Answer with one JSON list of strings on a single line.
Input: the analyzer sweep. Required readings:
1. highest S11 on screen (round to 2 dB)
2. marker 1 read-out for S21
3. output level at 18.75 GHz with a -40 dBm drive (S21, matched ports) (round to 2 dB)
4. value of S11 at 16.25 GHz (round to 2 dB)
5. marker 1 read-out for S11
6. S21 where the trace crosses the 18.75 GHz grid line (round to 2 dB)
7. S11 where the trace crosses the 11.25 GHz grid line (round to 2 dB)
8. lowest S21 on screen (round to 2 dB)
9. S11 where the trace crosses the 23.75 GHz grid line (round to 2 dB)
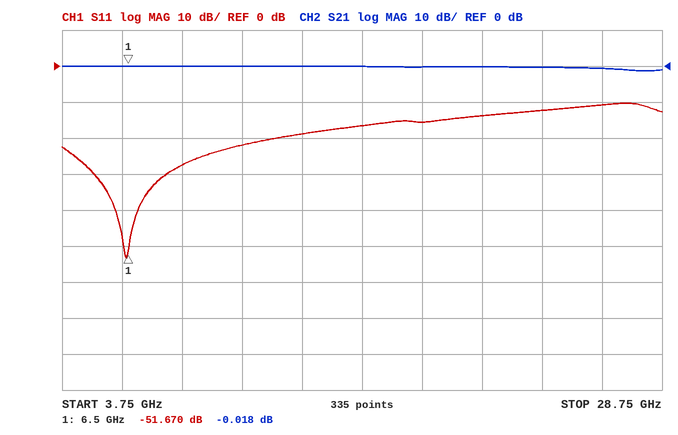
["-10 dB", "-0.018 dB", "-40 dBm", "-16 dB", "-51.670 dB", "0 dB", "-22 dB", "-2 dB", "-12 dB"]
